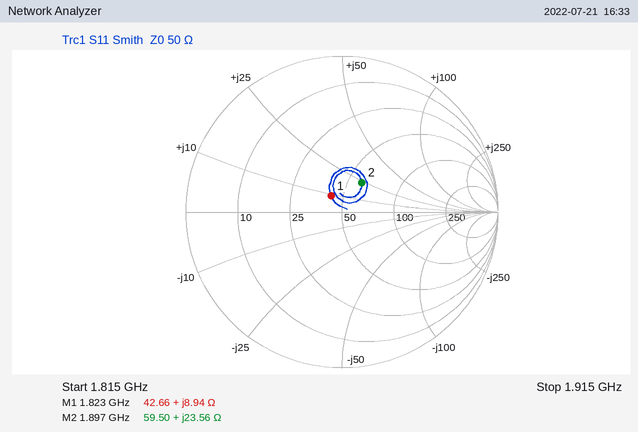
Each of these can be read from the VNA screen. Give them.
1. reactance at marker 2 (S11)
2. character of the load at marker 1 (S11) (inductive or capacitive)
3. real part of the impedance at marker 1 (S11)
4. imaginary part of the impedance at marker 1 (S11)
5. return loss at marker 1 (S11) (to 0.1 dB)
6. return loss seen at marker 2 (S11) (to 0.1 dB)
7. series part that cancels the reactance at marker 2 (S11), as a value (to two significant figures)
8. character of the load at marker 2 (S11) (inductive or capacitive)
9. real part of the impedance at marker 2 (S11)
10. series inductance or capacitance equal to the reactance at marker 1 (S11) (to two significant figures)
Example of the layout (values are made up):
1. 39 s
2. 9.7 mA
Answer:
1. +23.56 Ω
2. inductive
3. 42.66 Ω
4. +8.94 Ω
5. 18.1 dB
6. 12.9 dB
7. 3.6 pF
8. inductive
9. 59.50 Ω
10. 780 pH
